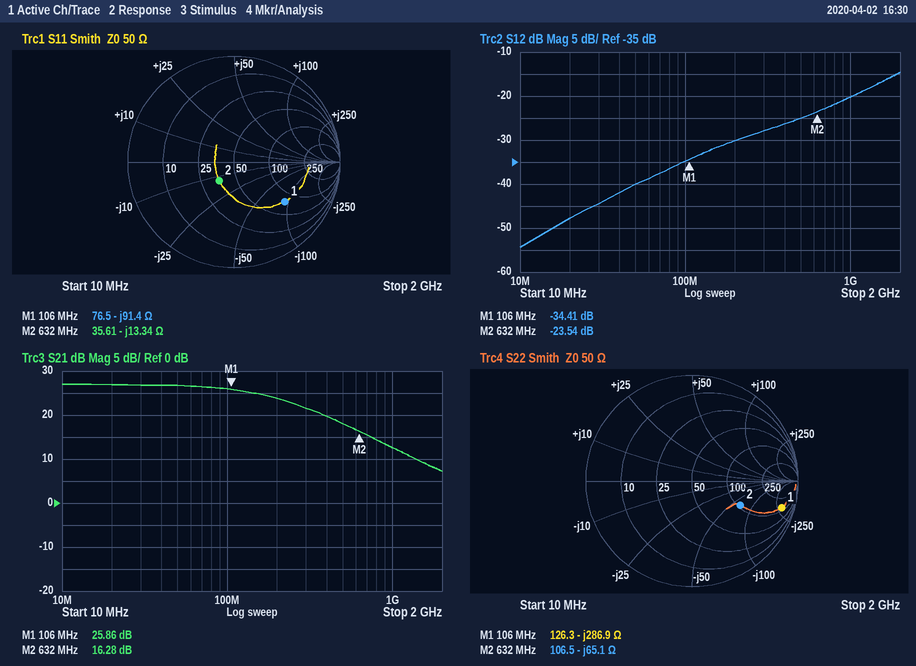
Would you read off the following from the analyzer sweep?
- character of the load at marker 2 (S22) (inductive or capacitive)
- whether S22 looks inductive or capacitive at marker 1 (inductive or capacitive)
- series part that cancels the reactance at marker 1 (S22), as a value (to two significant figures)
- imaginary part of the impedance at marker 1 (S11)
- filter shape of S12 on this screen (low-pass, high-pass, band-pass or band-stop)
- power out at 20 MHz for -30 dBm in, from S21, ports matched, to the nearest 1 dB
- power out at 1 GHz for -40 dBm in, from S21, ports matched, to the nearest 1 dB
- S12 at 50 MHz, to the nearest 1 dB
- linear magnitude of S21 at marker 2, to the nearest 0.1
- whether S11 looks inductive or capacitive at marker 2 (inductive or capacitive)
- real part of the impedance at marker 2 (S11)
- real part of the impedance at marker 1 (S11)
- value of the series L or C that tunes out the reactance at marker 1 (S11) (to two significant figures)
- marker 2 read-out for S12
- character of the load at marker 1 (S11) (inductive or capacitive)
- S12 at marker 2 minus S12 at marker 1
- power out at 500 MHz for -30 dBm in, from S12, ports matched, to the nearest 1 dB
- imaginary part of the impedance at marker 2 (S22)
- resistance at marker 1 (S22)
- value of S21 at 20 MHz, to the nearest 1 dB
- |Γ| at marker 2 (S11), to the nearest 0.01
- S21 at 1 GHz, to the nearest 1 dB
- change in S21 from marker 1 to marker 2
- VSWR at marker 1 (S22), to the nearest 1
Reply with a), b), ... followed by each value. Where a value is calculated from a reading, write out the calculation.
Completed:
a) capacitive
b) capacitive
c) L = 286.9 Ω/(2π × 106 MHz) ≈ 431 nH, so 430 nH to two significant figures
d) -91.4 Ω
e) high-pass
f) -30 dBm + (27 dB) = -3 dBm
g) -40 dBm + (13 dB) = -27 dBm
h) -40 dB
i) 10^(16.28/20) ≈ 6.5
j) capacitive
k) 35.61 Ω
l) 76.5 Ω
m) L = 91.4 Ω/(2π × 106 MHz) ≈ 137 nH, so 140 nH to two significant figures
n) -23.54 dB
o) capacitive
p) -23.54 − (-34.41) = 10.87 dB
q) -30 dBm + (-25 dB) = -55 dBm
r) -65.1 Ω
s) 126.3 Ω
t) 27 dB
u) 0.23
v) 13 dB
w) 16.28 − (25.86) = -9.58 dB
x) 16
